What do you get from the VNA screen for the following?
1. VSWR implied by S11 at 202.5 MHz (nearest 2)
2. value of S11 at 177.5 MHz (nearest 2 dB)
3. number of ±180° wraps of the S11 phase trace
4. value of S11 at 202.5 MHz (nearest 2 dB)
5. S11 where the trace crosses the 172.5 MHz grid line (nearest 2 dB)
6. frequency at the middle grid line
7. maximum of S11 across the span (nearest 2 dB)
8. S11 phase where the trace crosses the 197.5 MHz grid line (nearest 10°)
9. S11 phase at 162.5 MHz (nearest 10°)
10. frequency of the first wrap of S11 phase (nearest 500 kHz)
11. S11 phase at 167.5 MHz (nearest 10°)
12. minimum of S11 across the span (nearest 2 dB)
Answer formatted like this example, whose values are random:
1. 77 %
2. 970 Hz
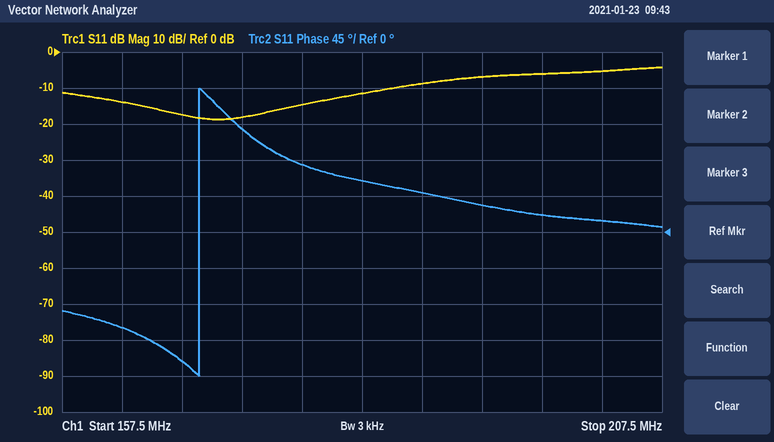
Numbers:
1. 4
2. -14 dB
3. 1
4. -6 dB
5. -18 dB
6. 182.5 MHz
7. -4 dB
8. 20°
9. -120°
10. 169.0 MHz
11. -160°
12. -18 dB
